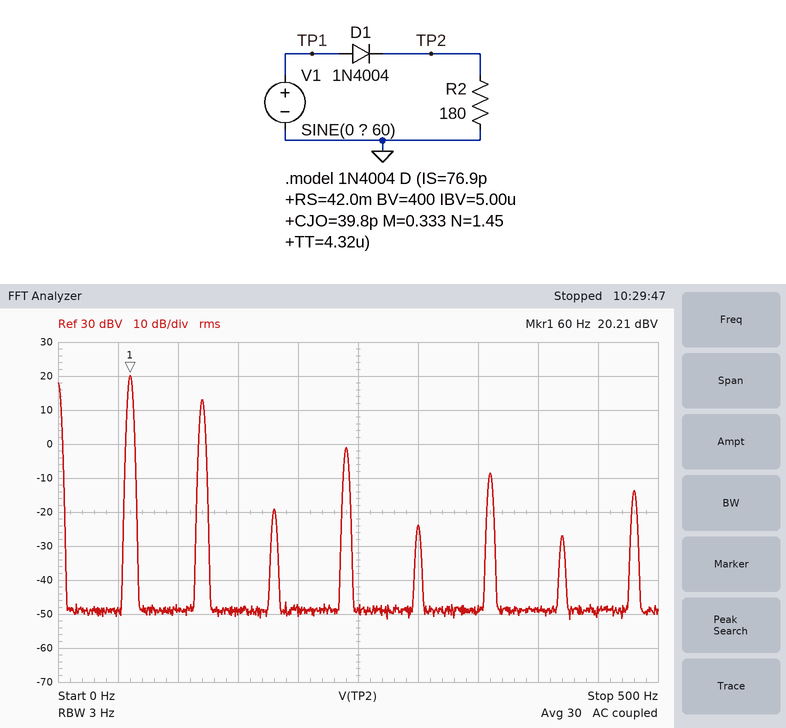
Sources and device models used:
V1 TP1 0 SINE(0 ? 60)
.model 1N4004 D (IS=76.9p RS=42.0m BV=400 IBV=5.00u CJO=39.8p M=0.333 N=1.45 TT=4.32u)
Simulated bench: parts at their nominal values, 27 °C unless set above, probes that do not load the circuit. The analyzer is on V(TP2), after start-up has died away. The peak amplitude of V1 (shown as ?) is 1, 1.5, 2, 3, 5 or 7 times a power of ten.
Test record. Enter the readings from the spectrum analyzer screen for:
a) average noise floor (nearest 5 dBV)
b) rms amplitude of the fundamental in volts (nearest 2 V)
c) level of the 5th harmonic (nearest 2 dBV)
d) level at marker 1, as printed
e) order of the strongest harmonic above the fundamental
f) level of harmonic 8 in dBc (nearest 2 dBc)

-50 dBV
10 V
-24 dBV
20.21 dBV
2
-34 dBc
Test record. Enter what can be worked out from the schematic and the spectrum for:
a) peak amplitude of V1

30 V
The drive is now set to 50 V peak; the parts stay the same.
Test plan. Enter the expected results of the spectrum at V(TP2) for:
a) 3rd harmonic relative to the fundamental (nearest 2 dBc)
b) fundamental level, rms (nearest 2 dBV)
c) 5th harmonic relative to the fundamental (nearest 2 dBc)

-44 dBc
24 dBV
-48 dBc
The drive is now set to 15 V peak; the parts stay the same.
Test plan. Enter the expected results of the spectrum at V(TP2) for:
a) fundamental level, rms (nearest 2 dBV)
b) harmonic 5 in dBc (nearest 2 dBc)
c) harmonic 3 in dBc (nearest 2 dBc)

14 dBV
-38 dBc
-34 dBc
